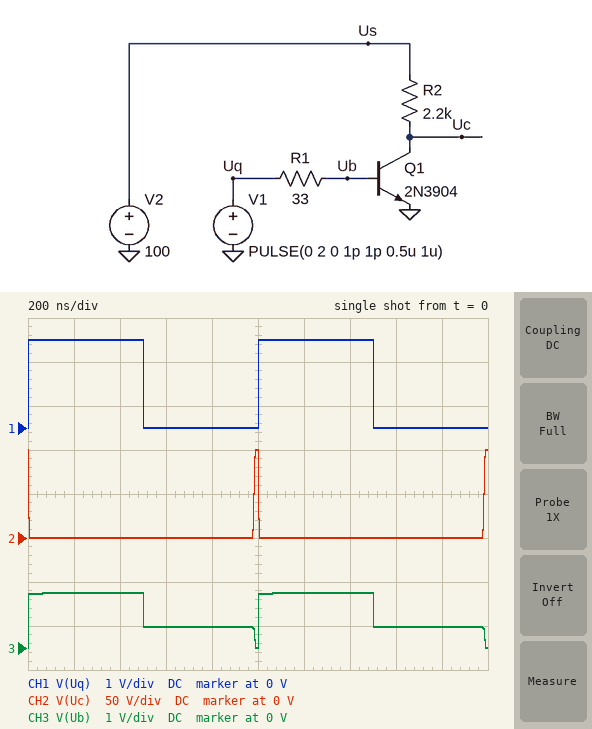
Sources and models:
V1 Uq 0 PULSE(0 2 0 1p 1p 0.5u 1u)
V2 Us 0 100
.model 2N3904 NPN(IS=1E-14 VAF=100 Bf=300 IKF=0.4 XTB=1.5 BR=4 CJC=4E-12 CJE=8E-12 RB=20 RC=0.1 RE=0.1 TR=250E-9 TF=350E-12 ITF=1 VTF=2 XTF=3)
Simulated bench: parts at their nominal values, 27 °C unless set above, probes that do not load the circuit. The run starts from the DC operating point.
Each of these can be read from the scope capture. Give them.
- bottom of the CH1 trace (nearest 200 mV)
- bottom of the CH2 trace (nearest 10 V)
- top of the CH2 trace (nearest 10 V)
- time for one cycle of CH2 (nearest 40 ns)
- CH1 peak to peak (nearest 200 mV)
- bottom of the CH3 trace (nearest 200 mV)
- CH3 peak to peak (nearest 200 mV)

0 V
0 V
100 V
1.00 µs
2.0 V
0 V
1.2 V
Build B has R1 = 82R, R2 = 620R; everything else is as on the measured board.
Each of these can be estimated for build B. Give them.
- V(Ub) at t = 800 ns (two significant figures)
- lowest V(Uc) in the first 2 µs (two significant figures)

650 mV
100 mV
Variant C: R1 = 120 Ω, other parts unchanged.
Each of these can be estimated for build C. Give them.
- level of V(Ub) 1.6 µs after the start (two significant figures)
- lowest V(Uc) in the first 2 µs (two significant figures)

650 mV
47 mV
